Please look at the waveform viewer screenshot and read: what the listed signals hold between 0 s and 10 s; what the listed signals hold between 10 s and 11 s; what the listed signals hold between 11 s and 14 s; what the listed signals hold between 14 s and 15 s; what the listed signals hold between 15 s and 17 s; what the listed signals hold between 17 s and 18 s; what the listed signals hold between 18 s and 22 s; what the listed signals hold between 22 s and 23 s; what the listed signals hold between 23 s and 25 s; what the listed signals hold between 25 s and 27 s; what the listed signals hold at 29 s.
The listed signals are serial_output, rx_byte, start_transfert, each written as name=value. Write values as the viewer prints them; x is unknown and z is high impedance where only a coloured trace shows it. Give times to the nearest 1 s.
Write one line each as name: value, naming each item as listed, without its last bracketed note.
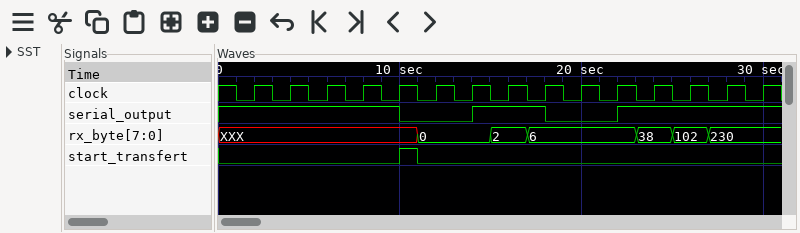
what the listed signals hold between 0 s and 10 s: serial_output=1, rx_byte=XXX, start_transfert=0
what the listed signals hold between 10 s and 11 s: serial_output=0, rx_byte=XXX, start_transfert=1
what the listed signals hold between 11 s and 14 s: serial_output=0, rx_byte=0, start_transfert=0
what the listed signals hold between 14 s and 15 s: serial_output=1, rx_byte=0, start_transfert=0
what the listed signals hold between 15 s and 17 s: serial_output=1, rx_byte=2, start_transfert=0
what the listed signals hold between 17 s and 18 s: serial_output=1, rx_byte=6, start_transfert=0
what the listed signals hold between 18 s and 22 s: serial_output=0, rx_byte=6, start_transfert=0
what the listed signals hold between 22 s and 23 s: serial_output=1, rx_byte=6, start_transfert=0
what the listed signals hold between 23 s and 25 s: serial_output=1, rx_byte=38, start_transfert=0
what the listed signals hold between 25 s and 27 s: serial_output=1, rx_byte=102, start_transfert=0
what the listed signals hold at 29 s: serial_output=1, rx_byte=230, start_transfert=0
